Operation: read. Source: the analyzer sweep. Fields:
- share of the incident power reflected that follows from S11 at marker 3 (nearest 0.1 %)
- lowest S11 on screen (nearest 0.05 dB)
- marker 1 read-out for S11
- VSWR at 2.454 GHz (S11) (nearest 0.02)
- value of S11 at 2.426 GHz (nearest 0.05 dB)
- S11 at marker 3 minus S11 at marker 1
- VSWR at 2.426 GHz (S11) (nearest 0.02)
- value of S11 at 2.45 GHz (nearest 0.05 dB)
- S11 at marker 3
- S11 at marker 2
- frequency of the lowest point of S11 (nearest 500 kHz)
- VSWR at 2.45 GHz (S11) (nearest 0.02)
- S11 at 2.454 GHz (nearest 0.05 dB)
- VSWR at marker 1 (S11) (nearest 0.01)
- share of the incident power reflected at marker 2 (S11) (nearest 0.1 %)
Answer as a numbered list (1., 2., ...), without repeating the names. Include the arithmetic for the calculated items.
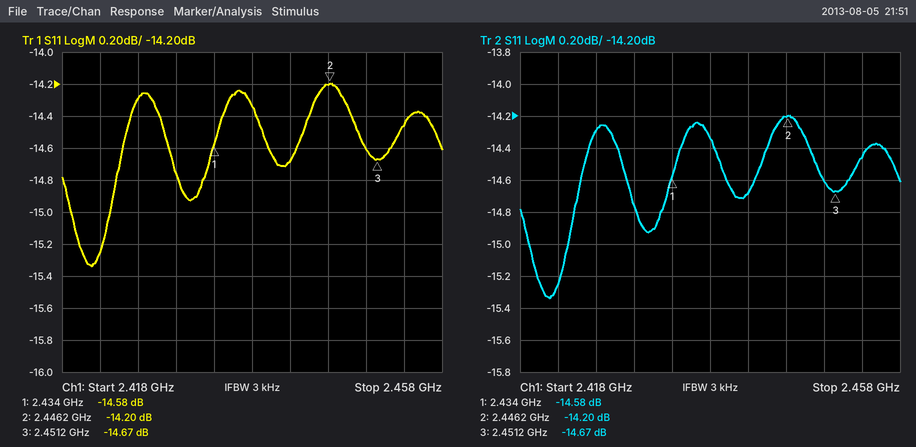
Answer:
1. 10^(-14.67/10) ≈ 3.4 %
2. -15.35 dB
3. -14.58 dB
4. |Γ| = 10^(-14.45/20) = 0.1895; VSWR = (1 + 0.1895)/(1 − 0.1895) ≈ 1.47, so 1.46 to the nearest 0.02
5. -14.30 dB
6. -14.67 − (-14.58) = -0.09 dB
7. |Γ| = 10^(-14.3/20) = 0.1928; VSWR = (1 + 0.1928)/(1 − 0.1928) ≈ 1.48
8. -14.60 dB
9. -14.67 dB
10. -14.20 dB
11. 2.4210 GHz
12. |Γ| = 10^(-14.6/20) = 0.1862; VSWR = (1 + 0.1862)/(1 − 0.1862) ≈ 1.46
13. -14.45 dB
14. (1 + 0.1866)/(1 − 0.1866) ≈ 1.46
15. 10^(-14.2/10) ≈ 3.8 %
